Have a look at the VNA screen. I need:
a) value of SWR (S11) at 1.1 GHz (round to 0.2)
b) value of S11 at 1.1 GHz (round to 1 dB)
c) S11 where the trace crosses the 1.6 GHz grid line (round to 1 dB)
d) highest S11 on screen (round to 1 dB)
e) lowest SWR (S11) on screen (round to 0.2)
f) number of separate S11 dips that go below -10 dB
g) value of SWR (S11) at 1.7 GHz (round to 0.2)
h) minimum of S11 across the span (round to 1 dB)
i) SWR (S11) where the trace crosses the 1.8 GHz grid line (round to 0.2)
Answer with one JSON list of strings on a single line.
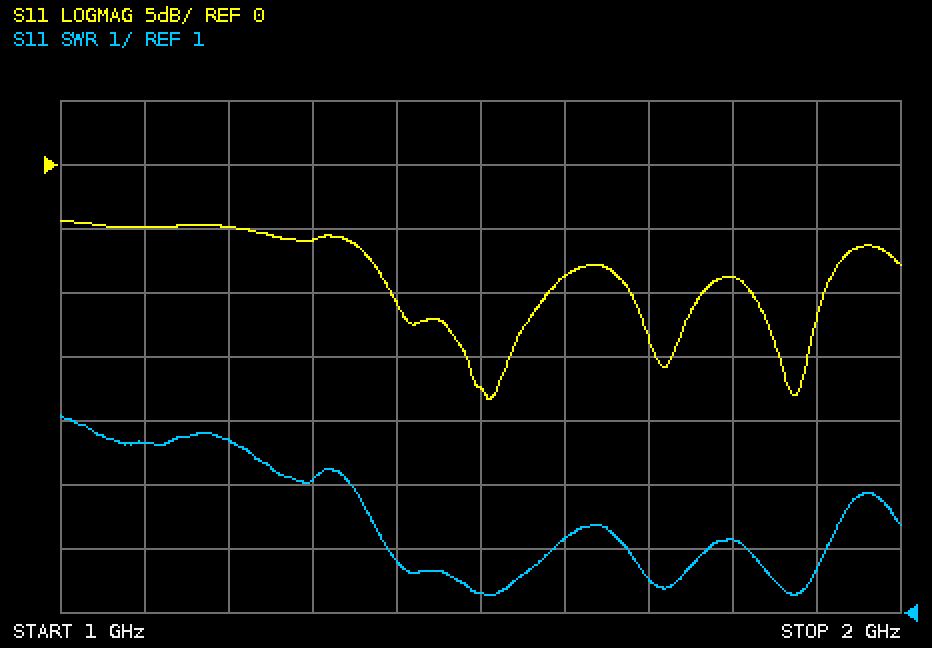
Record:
["3.6", "-5 dB", "-9 dB", "-4 dB", "1.2", "3", "1.6", "-18 dB", "2.2"]
